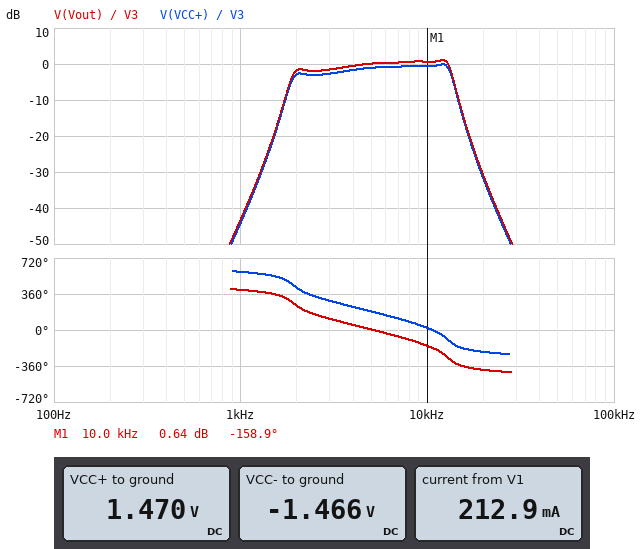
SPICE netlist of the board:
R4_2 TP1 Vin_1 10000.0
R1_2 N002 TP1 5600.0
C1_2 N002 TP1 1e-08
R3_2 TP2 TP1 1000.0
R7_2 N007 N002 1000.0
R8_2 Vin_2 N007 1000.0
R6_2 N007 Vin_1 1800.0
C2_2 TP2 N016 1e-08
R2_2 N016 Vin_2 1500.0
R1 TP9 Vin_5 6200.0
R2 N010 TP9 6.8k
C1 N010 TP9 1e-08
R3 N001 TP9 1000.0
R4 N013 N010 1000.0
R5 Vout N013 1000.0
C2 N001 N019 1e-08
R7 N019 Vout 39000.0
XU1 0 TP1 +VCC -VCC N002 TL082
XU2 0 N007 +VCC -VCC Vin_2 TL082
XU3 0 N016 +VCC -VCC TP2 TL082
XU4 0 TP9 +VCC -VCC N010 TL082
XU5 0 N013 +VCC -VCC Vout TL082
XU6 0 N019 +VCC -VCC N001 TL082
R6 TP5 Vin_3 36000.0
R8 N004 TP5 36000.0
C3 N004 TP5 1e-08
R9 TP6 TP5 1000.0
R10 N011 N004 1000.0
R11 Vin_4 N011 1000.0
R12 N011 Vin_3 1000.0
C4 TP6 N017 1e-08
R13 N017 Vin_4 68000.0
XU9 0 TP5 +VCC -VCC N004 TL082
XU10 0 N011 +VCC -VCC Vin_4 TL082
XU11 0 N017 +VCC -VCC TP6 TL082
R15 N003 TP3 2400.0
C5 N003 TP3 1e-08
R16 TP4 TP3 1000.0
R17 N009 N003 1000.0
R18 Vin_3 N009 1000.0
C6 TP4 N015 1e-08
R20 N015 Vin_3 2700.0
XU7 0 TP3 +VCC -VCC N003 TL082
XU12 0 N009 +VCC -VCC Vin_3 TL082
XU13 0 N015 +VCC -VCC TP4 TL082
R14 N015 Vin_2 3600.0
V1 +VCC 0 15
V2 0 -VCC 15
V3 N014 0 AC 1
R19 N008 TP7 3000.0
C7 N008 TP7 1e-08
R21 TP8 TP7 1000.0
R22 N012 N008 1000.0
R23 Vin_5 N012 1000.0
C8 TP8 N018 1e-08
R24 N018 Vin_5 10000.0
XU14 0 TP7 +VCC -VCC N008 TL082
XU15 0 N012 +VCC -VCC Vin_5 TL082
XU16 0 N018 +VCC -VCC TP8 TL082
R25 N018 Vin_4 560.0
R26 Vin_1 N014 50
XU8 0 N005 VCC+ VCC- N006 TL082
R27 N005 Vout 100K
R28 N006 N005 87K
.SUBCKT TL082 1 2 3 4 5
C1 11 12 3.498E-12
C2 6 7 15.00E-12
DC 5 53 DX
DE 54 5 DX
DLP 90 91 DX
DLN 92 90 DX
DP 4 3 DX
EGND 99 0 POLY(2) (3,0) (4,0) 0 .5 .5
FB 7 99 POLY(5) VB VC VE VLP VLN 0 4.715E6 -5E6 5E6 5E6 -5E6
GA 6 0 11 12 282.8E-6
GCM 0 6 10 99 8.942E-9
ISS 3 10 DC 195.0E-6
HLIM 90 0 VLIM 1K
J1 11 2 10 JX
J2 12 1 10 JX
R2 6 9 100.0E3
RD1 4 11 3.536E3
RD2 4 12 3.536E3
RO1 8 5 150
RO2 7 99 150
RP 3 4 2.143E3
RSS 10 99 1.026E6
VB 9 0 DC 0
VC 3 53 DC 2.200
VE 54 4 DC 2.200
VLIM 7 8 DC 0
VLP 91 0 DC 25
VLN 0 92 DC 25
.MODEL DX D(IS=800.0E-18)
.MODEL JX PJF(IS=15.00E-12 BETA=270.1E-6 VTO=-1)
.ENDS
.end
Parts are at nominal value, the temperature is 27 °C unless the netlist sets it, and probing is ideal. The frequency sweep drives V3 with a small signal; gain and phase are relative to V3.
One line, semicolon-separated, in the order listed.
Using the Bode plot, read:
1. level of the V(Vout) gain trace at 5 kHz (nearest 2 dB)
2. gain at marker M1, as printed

0 dB; 0.64 dB
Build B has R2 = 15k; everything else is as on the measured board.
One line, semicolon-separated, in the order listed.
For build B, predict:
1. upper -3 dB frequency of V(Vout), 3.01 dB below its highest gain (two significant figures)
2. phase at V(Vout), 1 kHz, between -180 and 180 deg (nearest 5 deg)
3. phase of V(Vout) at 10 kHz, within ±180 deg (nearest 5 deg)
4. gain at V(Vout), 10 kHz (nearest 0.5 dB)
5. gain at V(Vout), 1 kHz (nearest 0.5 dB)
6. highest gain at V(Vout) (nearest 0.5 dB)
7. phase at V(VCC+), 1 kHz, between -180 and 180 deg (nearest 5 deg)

3.7 kHz; 55 deg; -165 deg; 1.0 dB; -42.5 dB; 5.0 dB; -125 deg
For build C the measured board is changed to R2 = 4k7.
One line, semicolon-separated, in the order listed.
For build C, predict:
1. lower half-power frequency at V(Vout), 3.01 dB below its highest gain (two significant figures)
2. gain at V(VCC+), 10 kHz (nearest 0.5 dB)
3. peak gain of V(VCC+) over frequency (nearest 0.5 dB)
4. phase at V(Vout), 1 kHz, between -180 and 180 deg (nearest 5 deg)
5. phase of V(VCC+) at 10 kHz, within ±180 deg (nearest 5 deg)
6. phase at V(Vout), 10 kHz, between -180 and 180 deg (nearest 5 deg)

4.1 kHz; -1.0 dB; -0.5 dB; 35 deg; 25 deg; -155 deg
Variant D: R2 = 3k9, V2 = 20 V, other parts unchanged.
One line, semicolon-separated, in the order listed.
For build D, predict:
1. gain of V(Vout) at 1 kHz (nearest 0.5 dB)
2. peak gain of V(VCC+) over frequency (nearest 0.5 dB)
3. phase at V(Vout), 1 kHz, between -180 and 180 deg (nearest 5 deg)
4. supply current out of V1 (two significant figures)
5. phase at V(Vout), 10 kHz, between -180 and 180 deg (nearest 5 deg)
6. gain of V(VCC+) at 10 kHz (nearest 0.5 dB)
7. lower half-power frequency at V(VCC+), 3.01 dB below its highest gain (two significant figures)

-44.5 dB; -0.5 dB; 30 deg; 250 mA; -150 deg; -1.0 dB; 4.7 kHz
